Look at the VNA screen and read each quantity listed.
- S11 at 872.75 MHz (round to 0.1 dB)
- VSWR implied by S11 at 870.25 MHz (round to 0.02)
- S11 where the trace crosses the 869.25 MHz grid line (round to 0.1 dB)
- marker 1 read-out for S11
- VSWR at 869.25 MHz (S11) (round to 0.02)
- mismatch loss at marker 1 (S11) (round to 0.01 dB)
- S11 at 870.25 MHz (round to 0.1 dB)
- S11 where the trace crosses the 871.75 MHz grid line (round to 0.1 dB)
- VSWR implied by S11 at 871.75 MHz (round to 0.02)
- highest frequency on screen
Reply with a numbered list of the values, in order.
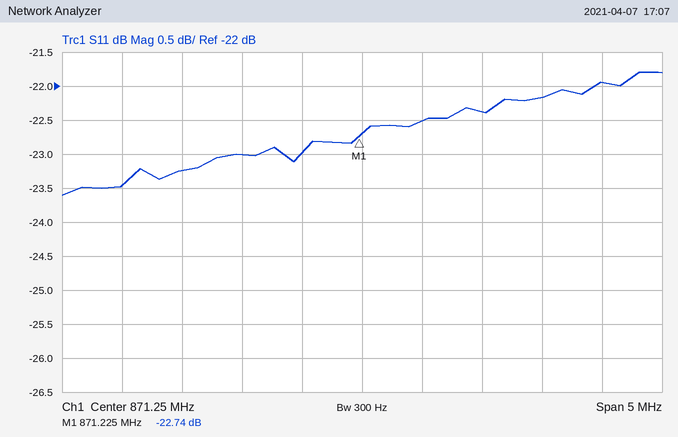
1. -22.2 dB
2. 1.16
3. -23.5 dB
4. -22.74 dB
5. 1.14
6. 0.02 dB
7. -23.0 dB
8. -22.5 dB
9. 1.16
10. 873.75 MHz
